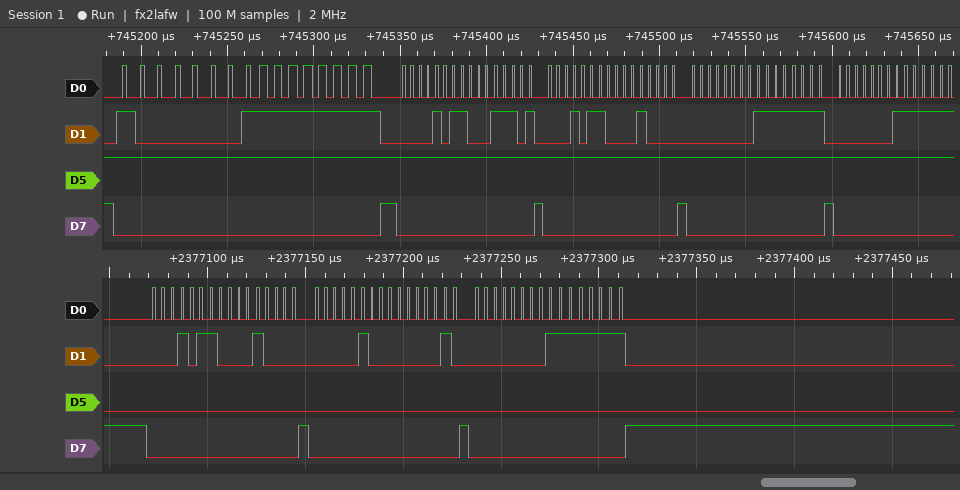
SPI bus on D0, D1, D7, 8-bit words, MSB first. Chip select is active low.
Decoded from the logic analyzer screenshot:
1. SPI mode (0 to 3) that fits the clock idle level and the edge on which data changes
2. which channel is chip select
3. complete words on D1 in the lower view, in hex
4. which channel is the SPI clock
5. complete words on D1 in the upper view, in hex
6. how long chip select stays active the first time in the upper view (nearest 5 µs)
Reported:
1
D7
16, 10, 04, 02, 00, FF
D0
81, FF, 0B, 1D, 16, 10, 00, FF, 01
155 µs
